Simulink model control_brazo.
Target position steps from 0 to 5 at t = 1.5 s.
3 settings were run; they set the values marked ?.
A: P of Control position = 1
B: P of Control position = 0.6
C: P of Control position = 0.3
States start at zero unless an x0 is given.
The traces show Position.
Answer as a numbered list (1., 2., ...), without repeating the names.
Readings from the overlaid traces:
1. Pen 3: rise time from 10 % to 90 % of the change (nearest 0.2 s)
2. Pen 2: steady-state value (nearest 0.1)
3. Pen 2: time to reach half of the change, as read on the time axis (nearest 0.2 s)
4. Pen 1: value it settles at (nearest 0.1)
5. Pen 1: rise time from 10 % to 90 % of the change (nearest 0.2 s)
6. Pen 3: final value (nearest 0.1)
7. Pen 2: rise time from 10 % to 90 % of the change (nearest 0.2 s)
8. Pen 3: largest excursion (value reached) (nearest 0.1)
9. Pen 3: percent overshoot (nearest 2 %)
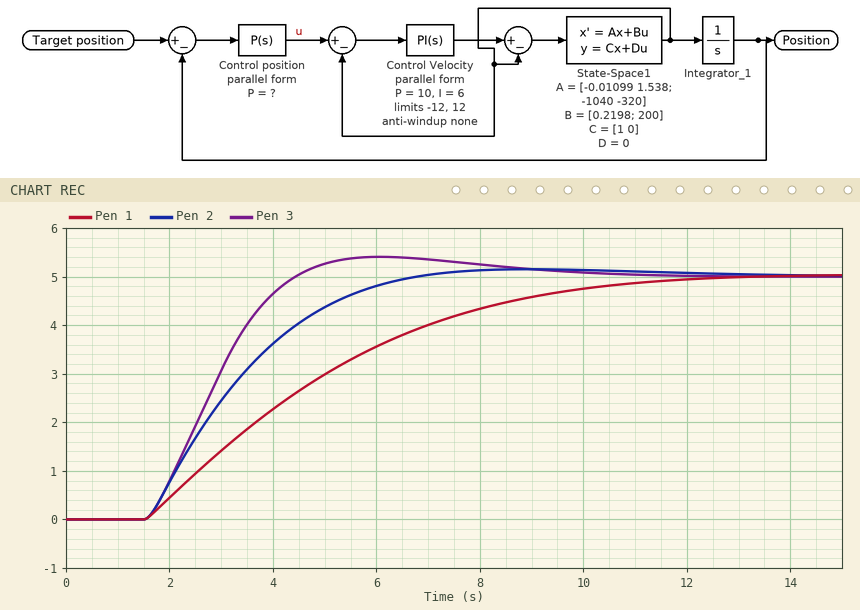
1. 2.0 s
2. 5.0
3. 3.0 s
4. 5.0
5. 6.6 s
6. 5.0
7. 3.4 s
8. 5.4
9. 8 %
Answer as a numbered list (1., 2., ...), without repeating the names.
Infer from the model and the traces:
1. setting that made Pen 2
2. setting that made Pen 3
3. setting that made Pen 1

1. B
2. A
3. C
